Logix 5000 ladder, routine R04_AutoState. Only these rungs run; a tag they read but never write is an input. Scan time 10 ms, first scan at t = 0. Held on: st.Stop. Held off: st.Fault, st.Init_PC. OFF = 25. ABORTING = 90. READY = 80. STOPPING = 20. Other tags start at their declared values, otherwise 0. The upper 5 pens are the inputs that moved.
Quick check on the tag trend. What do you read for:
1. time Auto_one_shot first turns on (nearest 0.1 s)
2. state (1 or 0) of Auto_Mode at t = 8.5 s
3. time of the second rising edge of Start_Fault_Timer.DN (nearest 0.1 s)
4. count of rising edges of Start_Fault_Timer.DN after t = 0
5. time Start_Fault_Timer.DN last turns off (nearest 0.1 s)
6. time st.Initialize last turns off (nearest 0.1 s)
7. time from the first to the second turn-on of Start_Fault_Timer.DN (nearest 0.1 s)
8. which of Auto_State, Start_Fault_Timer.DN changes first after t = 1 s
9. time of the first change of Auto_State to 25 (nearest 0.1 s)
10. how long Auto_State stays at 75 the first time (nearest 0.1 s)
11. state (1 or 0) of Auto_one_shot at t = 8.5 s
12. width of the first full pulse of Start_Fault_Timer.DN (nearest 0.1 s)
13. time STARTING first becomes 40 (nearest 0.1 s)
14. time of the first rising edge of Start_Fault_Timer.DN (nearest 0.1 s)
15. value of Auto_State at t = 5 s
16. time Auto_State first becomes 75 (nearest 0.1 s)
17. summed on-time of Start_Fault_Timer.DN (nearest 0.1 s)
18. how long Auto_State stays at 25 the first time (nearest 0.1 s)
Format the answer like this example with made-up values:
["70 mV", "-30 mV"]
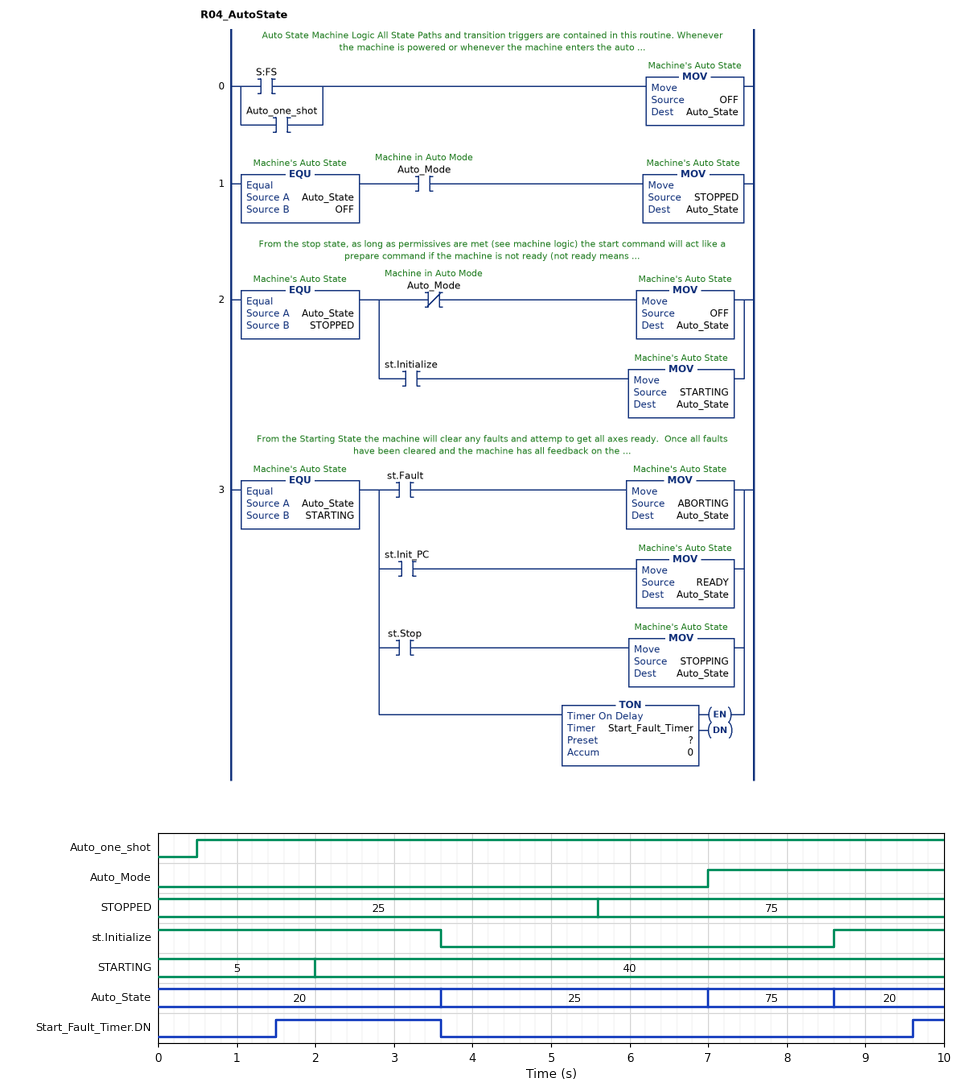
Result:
["0.5 s", "1", "9.6 s", "2", "3.6 s", "3.6 s", "8.1 s", "Start_Fault_Timer.DN", "3.6 s", "1.6 s", "1", "2.1 s", "2.0 s", "1.5 s", "25", "7.0 s", "2.5 s", "3.4 s"]
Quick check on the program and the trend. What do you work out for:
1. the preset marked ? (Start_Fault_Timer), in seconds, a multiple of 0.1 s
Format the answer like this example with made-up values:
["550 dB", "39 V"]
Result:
["1.0 s"]
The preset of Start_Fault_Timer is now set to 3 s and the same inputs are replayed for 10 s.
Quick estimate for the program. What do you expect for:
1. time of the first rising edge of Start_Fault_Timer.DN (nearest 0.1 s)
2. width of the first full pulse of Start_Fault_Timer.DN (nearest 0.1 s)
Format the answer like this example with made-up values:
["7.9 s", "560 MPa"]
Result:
["3.5 s", "0.1 s"]
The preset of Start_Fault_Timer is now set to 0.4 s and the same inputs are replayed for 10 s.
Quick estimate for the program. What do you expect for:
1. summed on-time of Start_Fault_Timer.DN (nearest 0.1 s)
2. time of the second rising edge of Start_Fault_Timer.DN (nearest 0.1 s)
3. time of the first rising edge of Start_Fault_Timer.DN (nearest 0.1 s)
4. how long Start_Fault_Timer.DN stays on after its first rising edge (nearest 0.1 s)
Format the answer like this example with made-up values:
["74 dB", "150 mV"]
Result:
["3.7 s", "9.0 s", "0.9 s", "2.7 s"]
